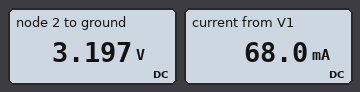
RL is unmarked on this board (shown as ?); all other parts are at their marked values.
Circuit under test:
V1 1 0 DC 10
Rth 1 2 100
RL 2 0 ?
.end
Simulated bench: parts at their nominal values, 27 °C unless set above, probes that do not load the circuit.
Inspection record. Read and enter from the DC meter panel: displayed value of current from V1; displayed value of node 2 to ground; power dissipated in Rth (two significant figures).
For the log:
68.0 mA
3.197 V
460 mW
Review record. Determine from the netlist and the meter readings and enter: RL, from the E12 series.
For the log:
47 Ω
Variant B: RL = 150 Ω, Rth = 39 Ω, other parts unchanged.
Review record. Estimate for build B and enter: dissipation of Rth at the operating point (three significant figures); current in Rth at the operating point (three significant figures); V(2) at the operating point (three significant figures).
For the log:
109 mW
52.9 mA
7.94 V
